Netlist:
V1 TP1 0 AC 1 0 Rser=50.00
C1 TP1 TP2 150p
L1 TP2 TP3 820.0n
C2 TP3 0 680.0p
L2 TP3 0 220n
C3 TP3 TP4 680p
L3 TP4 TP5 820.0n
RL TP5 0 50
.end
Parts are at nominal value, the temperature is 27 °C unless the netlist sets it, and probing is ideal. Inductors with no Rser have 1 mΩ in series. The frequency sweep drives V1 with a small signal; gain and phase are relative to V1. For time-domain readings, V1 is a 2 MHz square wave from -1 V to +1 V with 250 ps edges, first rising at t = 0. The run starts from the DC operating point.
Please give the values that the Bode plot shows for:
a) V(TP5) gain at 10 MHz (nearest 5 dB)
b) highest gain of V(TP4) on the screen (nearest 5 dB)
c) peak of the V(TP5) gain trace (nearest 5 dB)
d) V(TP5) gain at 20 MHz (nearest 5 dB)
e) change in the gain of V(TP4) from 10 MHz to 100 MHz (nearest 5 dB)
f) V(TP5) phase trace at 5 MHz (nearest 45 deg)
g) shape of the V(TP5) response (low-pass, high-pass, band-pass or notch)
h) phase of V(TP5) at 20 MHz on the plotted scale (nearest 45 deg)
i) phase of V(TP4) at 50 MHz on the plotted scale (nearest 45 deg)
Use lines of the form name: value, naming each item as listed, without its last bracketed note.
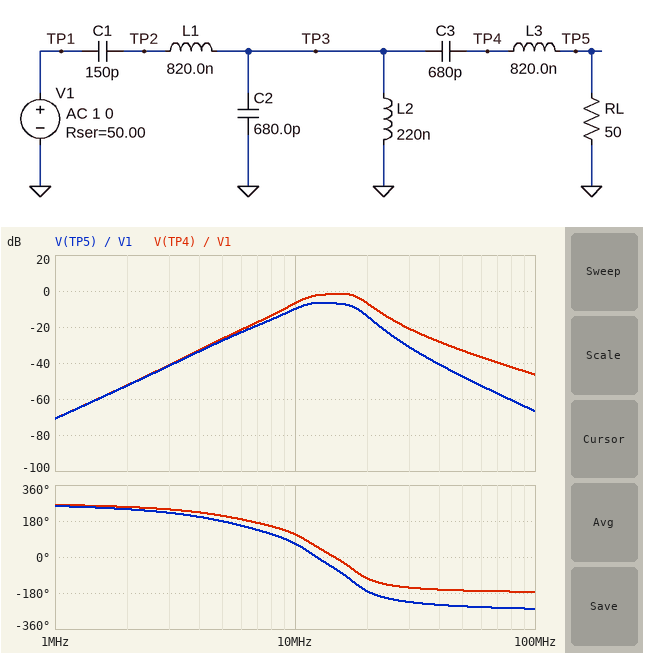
V(TP5) gain at 10 MHz: -10 dB
highest gain of V(TP4) on the screen: 0 dB
peak of the V(TP5) gain trace: -5 dB
V(TP5) gain at 20 MHz: -15 dB
change in the gain of V(TP4) from 10 MHz to 100 MHz: -40 dB
V(TP5) phase trace at 5 MHz: 180 deg
shape of the V(TP5) response: band-pass
phase of V(TP5) at 20 MHz on the plotted scale: -180 deg
phase of V(TP4) at 50 MHz on the plotted scale: -180 deg
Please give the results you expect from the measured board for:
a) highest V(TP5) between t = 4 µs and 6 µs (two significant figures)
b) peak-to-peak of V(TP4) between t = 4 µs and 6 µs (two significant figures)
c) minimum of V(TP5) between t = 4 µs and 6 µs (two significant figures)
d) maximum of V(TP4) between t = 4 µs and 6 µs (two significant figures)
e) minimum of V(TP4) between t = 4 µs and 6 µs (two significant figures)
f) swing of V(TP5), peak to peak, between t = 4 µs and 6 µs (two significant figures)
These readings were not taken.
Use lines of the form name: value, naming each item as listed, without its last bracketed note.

highest V(TP5) between t = 4 µs and 6 µs: 250 mV
peak-to-peak of V(TP4) between t = 4 µs and 6 µs: 830 mV
minimum of V(TP5) between t = 4 µs and 6 µs: -250 mV
maximum of V(TP4) between t = 4 µs and 6 µs: 420 mV
minimum of V(TP4) between t = 4 µs and 6 µs: -420 mV
swing of V(TP5), peak to peak, between t = 4 µs and 6 µs: 500 mV
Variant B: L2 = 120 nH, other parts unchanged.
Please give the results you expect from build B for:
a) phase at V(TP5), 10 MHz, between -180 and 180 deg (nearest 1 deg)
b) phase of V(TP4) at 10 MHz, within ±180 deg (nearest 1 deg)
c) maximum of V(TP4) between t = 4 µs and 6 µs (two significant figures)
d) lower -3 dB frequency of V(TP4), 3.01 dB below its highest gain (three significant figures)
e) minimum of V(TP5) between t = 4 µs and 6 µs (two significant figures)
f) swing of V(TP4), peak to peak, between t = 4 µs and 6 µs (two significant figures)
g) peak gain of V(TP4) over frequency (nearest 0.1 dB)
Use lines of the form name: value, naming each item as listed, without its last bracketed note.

phase at V(TP5), 10 MHz, between -180 and 180 deg: 93 deg
phase of V(TP4) at 10 MHz, within ±180 deg: 139 deg
maximum of V(TP4) between t = 4 µs and 6 µs: 330 mV
lower -3 dB frequency of V(TP4), 3.01 dB below its highest gain: 18.0 MHz
minimum of V(TP5) between t = 4 µs and 6 µs: -180 mV
swing of V(TP4), peak to peak, between t = 4 µs and 6 µs: 660 mV
peak gain of V(TP4) over frequency: 0.5 dB
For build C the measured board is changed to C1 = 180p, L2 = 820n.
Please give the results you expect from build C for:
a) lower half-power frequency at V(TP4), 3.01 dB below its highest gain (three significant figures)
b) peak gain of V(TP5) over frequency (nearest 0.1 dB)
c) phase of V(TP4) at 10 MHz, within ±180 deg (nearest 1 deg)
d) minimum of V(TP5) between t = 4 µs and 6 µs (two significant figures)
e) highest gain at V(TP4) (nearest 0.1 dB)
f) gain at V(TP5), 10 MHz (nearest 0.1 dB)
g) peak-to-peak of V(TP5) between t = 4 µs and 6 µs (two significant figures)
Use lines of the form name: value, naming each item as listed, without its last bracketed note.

lower half-power frequency at V(TP4), 3.01 dB below its highest gain: 5.85 MHz
peak gain of V(TP5) over frequency: -8.3 dB
phase of V(TP4) at 10 MHz, within ±180 deg: 12 deg
minimum of V(TP5) between t = 4 µs and 6 µs: -280 mV
highest gain at V(TP4): -5.1 dB
gain at V(TP5), 10 MHz: -8.5 dB
peak-to-peak of V(TP5) between t = 4 µs and 6 µs: 560 mV
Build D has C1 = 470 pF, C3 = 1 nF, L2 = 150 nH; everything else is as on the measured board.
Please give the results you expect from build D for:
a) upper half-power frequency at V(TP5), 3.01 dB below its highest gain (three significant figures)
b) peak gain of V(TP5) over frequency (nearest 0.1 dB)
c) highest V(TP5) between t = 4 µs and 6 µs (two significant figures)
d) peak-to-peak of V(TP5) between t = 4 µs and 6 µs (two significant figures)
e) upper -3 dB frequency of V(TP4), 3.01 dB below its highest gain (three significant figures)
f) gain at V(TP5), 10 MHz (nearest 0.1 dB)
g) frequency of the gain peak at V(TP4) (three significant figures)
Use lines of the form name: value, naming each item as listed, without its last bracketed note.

upper half-power frequency at V(TP5), 3.01 dB below its highest gain: 19.3 MHz
peak gain of V(TP5) over frequency: -6.1 dB
highest V(TP5) between t = 4 µs and 6 µs: 210 mV
peak-to-peak of V(TP5) between t = 4 µs and 6 µs: 420 mV
upper -3 dB frequency of V(TP4), 3.01 dB below its highest gain: 19.4 MHz
gain at V(TP5), 10 MHz: -14.9 dB
frequency of the gain peak at V(TP4): 18.1 MHz
